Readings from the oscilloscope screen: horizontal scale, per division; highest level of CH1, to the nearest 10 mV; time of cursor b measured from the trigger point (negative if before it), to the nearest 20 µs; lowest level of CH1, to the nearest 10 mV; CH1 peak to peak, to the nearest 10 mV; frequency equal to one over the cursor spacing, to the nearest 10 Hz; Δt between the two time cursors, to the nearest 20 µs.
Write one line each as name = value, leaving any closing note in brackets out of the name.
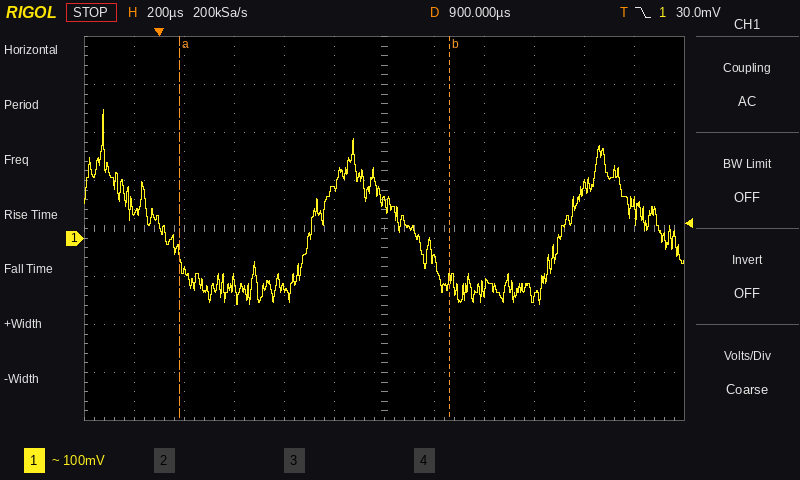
horizontal scale, per division = 200 µs
highest level of CH1, to the nearest 10 mV = 270 mV
time of cursor b measured from the trigger point (negative if before it), to the nearest 20 µs = +1.16 ms
lowest level of CH1, to the nearest 10 mV = -140 mV
CH1 peak to peak, to the nearest 10 mV = 410 mV
frequency equal to one over the cursor spacing, to the nearest 10 Hz = 930 Hz
Δt between the two time cursors, to the nearest 20 µs = 1.08 ms
